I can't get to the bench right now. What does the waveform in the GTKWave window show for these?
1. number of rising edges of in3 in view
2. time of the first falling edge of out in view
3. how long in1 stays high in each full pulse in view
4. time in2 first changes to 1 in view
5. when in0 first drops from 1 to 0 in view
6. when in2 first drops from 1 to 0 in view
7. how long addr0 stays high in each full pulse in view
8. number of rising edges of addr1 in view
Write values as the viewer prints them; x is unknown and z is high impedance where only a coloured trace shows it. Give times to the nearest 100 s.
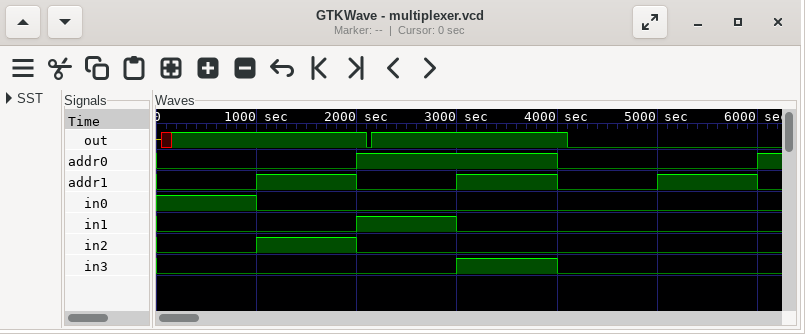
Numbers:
1
2100 s
1000 s
1000 s
1000 s
2000 s
2000 s
3
